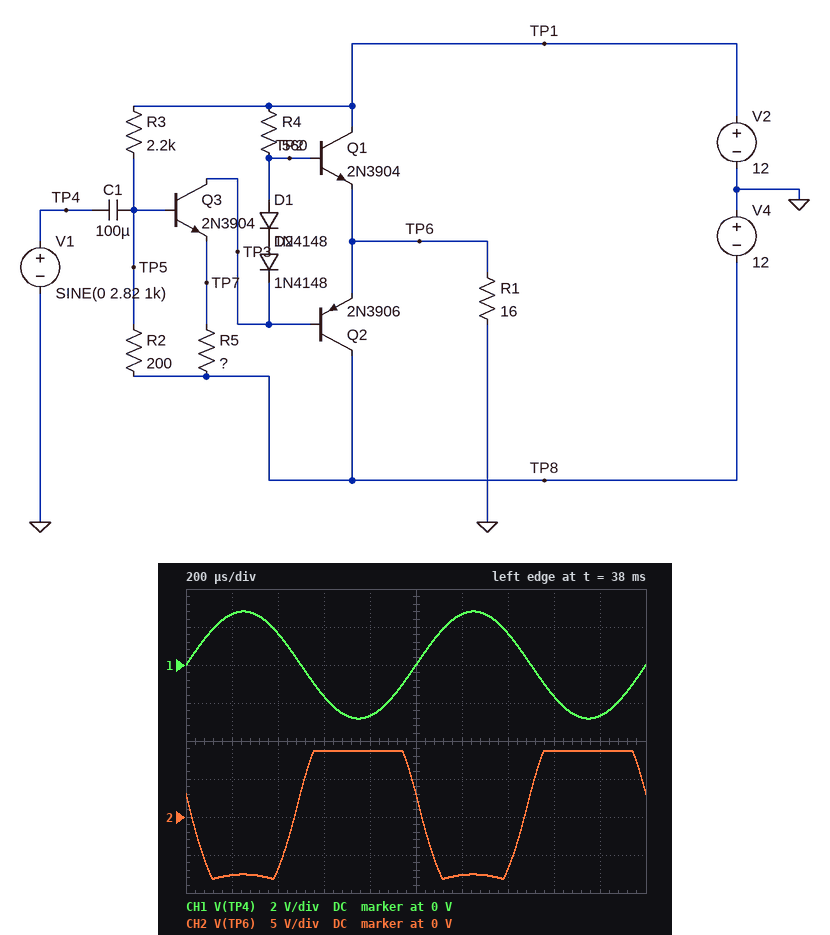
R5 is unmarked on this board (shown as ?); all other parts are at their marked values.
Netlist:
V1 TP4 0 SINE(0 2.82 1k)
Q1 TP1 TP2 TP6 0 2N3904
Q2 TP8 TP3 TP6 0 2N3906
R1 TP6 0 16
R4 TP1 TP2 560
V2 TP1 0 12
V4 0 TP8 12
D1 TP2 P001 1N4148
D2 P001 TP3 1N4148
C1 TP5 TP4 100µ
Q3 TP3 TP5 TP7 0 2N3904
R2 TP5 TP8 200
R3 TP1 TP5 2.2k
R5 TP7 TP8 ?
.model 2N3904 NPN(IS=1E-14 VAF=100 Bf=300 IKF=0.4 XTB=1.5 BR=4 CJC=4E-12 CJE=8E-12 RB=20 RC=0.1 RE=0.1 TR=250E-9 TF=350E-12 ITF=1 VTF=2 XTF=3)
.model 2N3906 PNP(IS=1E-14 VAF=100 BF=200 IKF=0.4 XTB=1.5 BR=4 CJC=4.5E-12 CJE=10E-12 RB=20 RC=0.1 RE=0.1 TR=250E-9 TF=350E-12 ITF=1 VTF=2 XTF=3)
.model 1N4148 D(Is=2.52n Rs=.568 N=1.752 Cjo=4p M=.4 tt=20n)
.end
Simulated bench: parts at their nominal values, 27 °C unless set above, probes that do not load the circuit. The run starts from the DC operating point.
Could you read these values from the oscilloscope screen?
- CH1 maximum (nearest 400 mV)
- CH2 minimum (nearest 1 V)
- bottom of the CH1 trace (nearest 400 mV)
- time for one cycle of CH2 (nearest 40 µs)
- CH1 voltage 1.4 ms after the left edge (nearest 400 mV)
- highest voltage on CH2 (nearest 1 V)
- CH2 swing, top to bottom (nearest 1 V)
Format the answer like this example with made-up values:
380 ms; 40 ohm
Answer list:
2.8 V; -8 V; -2.8 V; 1.00 ms; 1.6 V; 9 V; 17 V
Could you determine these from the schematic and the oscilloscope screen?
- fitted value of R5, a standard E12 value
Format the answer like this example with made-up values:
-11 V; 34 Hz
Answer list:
68 Ω
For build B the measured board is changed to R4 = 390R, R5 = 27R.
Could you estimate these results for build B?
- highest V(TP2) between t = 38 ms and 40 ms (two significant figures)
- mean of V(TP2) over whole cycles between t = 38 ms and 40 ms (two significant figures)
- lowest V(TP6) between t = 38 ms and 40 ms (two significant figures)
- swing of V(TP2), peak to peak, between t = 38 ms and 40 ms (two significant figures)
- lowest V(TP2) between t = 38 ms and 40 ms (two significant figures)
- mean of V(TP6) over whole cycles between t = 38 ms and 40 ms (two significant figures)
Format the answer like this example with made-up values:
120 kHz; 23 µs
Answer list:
10 V; 2.3 V; -9.2 V; 19 V; -8.7 V; 1.5 V
